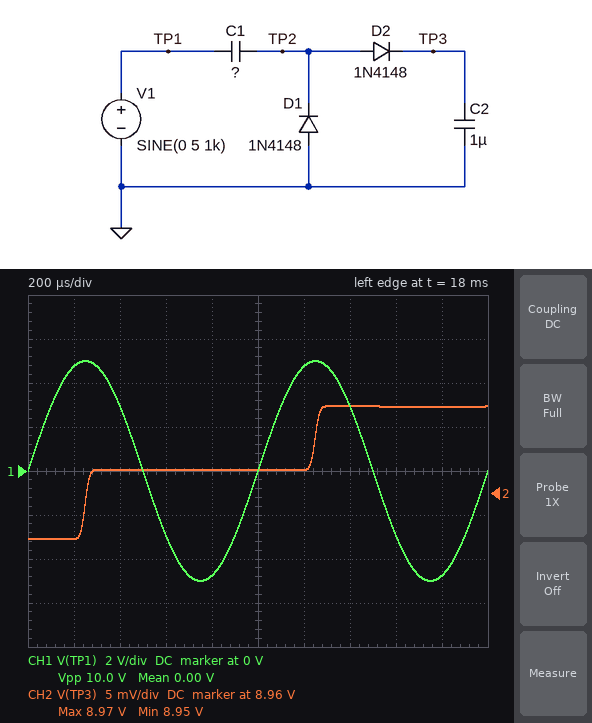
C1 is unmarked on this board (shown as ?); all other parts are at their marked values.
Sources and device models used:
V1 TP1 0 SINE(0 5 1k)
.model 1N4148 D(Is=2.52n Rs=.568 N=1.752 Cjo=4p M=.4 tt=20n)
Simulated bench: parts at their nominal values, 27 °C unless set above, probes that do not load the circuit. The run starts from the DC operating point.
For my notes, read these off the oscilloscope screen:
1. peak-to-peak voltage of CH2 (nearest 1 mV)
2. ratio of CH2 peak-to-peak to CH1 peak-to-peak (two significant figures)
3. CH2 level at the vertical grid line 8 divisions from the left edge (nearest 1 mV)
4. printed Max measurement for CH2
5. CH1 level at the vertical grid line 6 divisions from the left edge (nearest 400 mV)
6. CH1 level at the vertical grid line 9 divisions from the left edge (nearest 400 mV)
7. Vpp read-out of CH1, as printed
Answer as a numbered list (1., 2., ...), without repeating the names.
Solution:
1. 15 mV
2. 0.0015
3. 8.970 V
4. 8.97 V
5. 4.8 V
6. -4.8 V
7. 10.0 V
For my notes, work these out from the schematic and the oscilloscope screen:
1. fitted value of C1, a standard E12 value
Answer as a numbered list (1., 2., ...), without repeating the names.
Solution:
1. 820 nF
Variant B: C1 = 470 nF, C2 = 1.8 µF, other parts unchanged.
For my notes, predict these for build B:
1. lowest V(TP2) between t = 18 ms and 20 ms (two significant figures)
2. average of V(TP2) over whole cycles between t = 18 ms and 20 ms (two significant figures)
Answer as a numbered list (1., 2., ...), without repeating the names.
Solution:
1. -600 mV
2. 4.4 V
